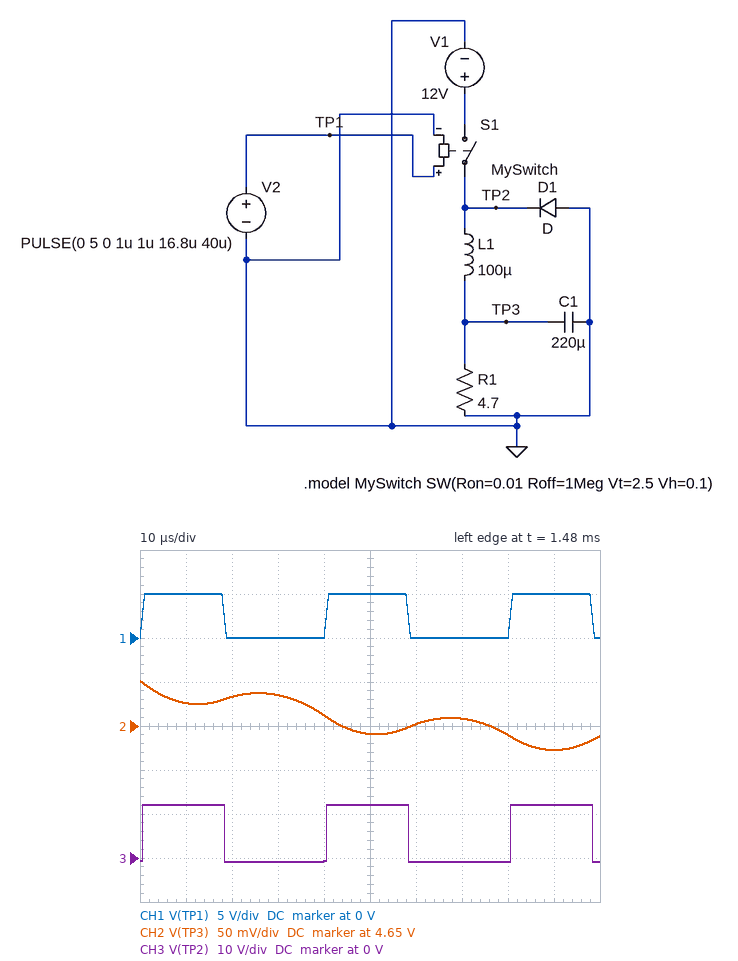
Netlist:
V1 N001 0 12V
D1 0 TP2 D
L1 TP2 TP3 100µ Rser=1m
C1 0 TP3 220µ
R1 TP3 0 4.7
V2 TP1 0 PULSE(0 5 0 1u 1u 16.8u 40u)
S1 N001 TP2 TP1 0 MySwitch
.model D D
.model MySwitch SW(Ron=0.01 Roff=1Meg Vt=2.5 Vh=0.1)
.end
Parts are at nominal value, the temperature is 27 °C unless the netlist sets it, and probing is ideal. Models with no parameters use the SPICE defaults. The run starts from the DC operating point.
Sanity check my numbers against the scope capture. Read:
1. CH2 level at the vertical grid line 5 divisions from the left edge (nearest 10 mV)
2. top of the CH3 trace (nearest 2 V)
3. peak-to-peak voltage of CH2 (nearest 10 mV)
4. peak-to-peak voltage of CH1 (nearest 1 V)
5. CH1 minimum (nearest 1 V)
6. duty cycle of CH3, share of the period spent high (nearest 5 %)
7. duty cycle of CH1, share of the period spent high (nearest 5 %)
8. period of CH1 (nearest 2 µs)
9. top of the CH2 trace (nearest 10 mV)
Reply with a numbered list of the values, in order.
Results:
1. 4.64 V
2. 12 V
3. 80 mV
4. 5 V
5. 0 V
6. 45 %
7. 45 %
8. 40 µs
9. 4.70 V
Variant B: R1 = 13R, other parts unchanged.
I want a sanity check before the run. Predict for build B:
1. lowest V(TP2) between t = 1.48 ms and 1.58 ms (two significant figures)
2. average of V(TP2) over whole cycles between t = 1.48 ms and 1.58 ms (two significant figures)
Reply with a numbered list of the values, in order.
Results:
1. -830 mV
2. 7.3 V
